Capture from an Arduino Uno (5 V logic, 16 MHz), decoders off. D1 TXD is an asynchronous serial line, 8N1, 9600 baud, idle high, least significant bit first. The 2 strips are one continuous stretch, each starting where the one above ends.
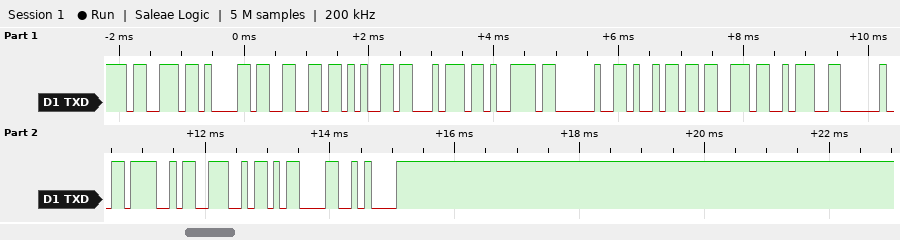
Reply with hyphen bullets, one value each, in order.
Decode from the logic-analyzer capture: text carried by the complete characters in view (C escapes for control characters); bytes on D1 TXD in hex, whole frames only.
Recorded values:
- "safety is: ON\r\n"
- 73 61 66 65 74 79 20 69 73 3A 20 4F 4E 0D 0A
